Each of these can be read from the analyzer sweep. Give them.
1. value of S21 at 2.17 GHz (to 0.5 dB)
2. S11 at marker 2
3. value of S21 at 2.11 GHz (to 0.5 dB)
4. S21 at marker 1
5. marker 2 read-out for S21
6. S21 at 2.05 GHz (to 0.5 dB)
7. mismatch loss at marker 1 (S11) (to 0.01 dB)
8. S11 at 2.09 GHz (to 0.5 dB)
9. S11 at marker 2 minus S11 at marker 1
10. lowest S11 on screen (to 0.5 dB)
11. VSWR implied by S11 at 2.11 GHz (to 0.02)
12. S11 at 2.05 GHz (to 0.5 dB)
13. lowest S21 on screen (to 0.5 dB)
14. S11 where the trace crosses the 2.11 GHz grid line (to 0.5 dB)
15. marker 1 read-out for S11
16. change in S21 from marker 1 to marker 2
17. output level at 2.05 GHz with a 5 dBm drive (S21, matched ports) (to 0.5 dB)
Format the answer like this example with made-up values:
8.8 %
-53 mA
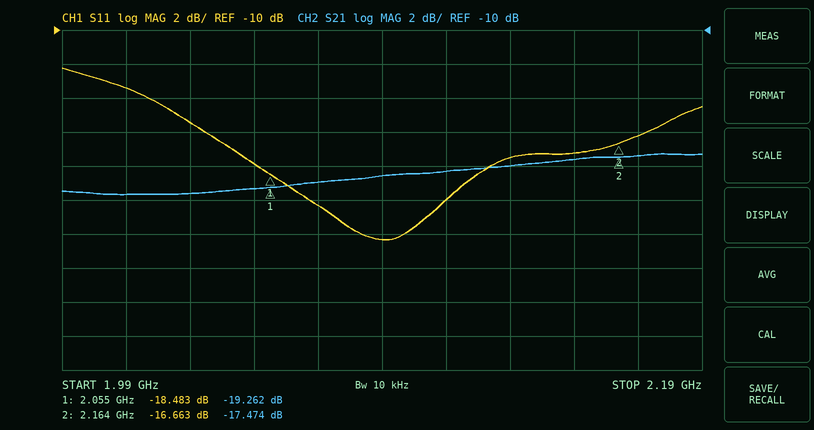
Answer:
-17.5 dB
-16.663 dB
-18.5 dB
-19.262 dB
-17.474 dB
-19.5 dB
0.06 dB
-22.5 dB
1.820 dB
-22.5 dB
1.22
-18.0 dB
-19.5 dB
-20.0 dB
-18.483 dB
1.788 dB
-14.5 dBm
